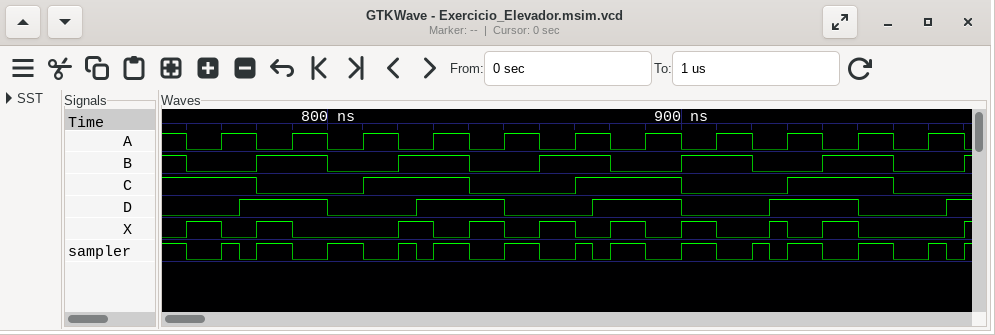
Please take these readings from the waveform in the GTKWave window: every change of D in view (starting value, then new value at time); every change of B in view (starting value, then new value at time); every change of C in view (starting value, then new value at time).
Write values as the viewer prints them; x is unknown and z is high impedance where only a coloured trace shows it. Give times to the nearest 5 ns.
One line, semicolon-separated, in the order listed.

0, 1 at 775 ns, 0 at 800 ns, 1 at 825 ns, 0 at 850 ns, 1 at 875 ns, 0 at 900 ns, 1 at 925 ns, 0 at 950 ns, 1 at 975 ns; 1, 0 at 760 ns, 1 at 780 ns, 0 at 800 ns, 1 at 820 ns, 0 at 840 ns, 1 at 860 ns, 0 at 880 ns, 1 at 900 ns, 0 at 920 ns, 1 at 940 ns, 0 at 960 ns, 1 at 980 ns; 1, 0 at 780 ns, 1 at 810 ns, 0 at 840 ns, 1 at 870 ns, 0 at 900 ns, 1 at 930 ns, 0 at 960 ns
